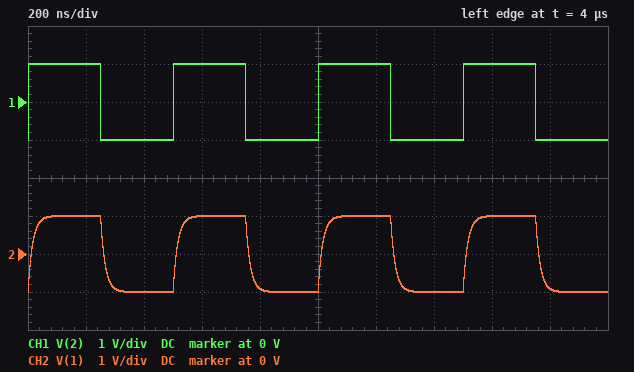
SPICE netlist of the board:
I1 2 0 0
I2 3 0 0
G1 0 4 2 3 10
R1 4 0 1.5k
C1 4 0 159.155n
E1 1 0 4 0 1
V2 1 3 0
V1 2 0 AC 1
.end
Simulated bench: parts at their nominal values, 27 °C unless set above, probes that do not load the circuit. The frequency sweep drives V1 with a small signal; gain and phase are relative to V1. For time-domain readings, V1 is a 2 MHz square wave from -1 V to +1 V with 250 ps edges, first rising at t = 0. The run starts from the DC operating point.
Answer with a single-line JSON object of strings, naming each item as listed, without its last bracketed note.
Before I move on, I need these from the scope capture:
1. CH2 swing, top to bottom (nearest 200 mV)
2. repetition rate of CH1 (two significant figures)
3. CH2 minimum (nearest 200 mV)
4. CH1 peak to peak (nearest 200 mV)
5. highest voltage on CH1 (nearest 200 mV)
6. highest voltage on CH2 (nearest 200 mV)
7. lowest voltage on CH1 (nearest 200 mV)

{"CH2 swing, top to bottom": "2.0 V", "repetition rate of CH1": "2.0 MHz", "CH2 minimum": "-1.0 V", "CH1 peak to peak": "2.0 V", "highest voltage on CH1": "1.0 V", "highest voltage on CH2": "1.0 V", "lowest voltage on CH1": "-1.0 V"}
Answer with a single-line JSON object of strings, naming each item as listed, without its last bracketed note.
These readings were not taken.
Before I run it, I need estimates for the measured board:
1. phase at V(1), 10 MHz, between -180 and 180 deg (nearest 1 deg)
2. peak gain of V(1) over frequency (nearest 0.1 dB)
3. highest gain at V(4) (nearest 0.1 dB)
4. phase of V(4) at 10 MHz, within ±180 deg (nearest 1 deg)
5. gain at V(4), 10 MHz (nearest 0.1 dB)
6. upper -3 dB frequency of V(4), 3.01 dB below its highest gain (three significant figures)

{"phase at V(1), 10 MHz, between -180 and 180 deg": "-45 deg", "peak gain of V(1) over frequency": "0 dB", "highest gain at V(4)": "0 dB", "phase of V(4) at 10 MHz, within ±180 deg": "-45 deg", "gain at V(4), 10 MHz": "-3.0 dB", "upper -3 dB frequency of V(4), 3.01 dB below its highest gain": "10.0 MHz"}
